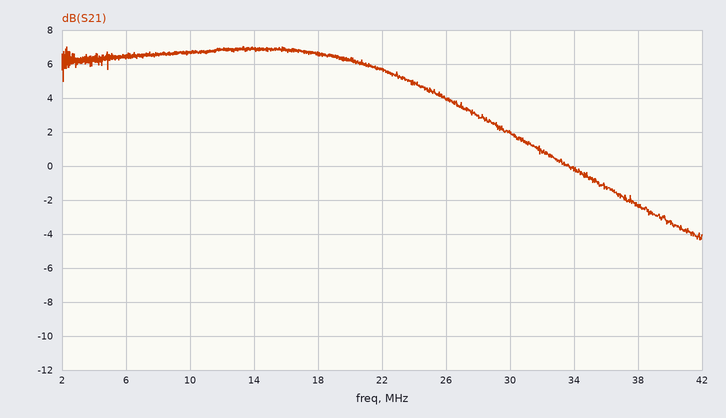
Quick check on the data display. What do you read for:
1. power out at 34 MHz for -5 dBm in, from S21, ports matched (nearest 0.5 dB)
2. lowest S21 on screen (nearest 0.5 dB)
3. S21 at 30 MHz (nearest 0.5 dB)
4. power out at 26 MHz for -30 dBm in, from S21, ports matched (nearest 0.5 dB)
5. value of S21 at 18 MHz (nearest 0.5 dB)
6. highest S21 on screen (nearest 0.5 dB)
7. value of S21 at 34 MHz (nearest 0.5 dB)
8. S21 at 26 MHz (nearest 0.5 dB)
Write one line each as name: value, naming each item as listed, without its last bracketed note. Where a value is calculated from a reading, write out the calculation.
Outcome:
power out at 34 MHz for -5 dBm in, from S21, ports matched: -5 dBm + (0.0 dB) = -5.0 dBm
lowest S21 on screen: -4.5 dB
S21 at 30 MHz: 2.0 dB
power out at 26 MHz for -30 dBm in, from S21, ports matched: -30 dBm + (4.0 dB) = -26.0 dBm
value of S21 at 18 MHz: 6.5 dB
highest S21 on screen: 7.0 dB
value of S21 at 34 MHz: 0.0 dB
S21 at 26 MHz: 4.0 dB
